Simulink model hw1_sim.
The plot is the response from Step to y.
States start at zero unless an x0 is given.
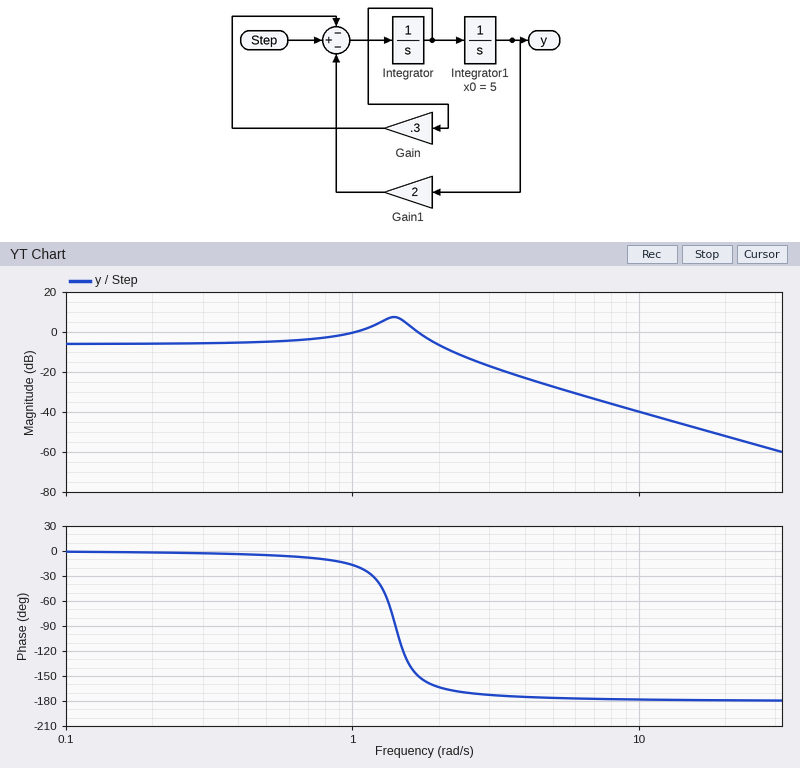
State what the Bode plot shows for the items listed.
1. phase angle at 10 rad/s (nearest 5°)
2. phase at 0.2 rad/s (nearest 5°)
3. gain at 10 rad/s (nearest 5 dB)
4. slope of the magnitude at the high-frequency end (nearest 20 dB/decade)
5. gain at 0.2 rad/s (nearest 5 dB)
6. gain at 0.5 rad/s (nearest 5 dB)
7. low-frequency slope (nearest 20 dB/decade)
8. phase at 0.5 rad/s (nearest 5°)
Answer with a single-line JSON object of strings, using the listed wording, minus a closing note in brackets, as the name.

{"phase angle at 10 rad/s": "-180°", "phase at 0.2 rad/s": "0°", "gain at 10 rad/s": "-40 dB", "slope of the magnitude at the high-frequency end": "-40 dB/decade", "gain at 0.2 rad/s": "-5 dB", "gain at 0.5 rad/s": "-5 dB", "low-frequency slope": "0 dB/decade", "phase at 0.5 rad/s": "-5°"}
